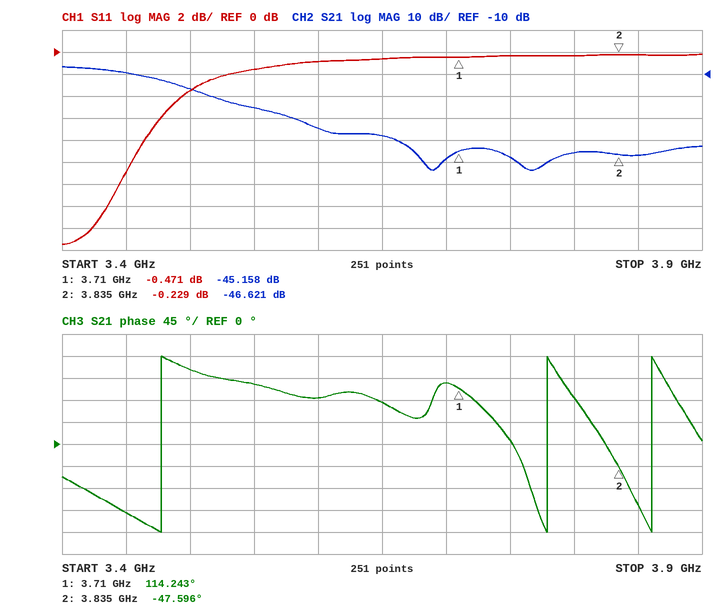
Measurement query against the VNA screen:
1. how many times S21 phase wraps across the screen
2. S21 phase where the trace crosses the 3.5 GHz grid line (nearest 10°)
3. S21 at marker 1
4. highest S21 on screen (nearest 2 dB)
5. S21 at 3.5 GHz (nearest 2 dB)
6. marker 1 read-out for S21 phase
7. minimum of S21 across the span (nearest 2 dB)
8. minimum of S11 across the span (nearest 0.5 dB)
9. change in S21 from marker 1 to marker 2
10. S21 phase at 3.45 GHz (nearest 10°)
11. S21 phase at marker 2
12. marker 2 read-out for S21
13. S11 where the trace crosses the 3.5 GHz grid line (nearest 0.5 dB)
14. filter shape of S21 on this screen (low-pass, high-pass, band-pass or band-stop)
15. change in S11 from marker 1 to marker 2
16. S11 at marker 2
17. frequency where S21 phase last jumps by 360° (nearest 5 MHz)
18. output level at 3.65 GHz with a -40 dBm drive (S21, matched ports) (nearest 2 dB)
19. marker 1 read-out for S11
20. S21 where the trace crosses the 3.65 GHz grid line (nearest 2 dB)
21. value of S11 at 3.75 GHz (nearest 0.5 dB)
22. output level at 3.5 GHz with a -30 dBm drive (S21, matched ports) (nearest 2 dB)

3
150°
-45.158 dB
-6 dB
-16 dB
114.243°
-54 dB
-17.5 dB
-1.463 dB
-140°
-47.596°
-46.621 dB
-3.5 dB
low-pass
0.242 dB
-0.229 dB
3.860 GHz
-78 dBm
-0.471 dB
-38 dB
-0.5 dB
-46 dBm
